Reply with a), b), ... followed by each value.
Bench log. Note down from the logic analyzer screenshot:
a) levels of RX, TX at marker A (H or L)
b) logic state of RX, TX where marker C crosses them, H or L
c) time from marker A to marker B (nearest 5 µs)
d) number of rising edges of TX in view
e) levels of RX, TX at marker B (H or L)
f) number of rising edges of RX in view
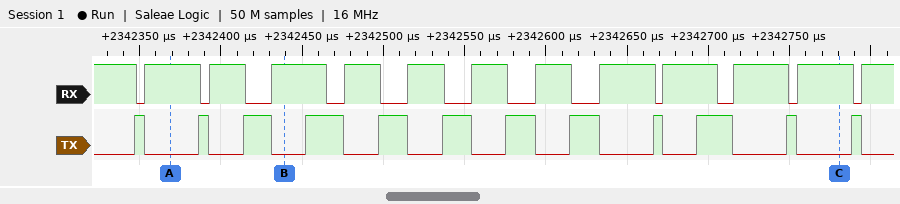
a) RX=H, TX=L
b) RX=H, TX=L
c) 70 µs
d) 12
e) RX=H, TX=L
f) 12
